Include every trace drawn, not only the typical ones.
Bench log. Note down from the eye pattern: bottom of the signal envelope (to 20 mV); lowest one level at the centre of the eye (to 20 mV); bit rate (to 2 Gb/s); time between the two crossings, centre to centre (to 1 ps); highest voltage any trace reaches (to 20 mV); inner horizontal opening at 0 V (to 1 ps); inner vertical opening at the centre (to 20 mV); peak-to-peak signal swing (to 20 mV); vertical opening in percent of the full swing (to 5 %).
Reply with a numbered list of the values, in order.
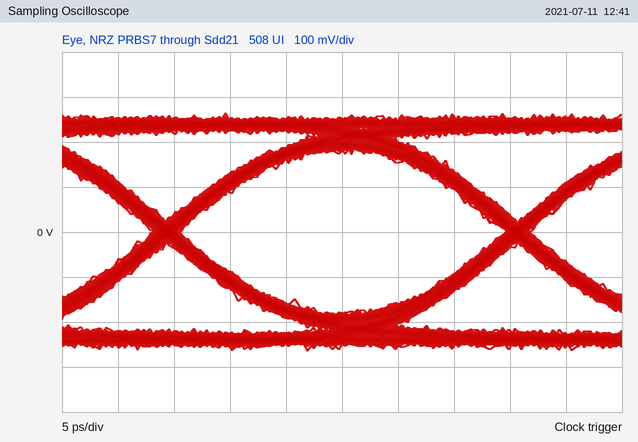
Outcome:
1. -260 mV
2. 180 mV
3. 32 Gb/s
4. 31 ps
5. 260 mV
6. 29 ps
7. 360 mV
8. 520 mV
9. 70 %
